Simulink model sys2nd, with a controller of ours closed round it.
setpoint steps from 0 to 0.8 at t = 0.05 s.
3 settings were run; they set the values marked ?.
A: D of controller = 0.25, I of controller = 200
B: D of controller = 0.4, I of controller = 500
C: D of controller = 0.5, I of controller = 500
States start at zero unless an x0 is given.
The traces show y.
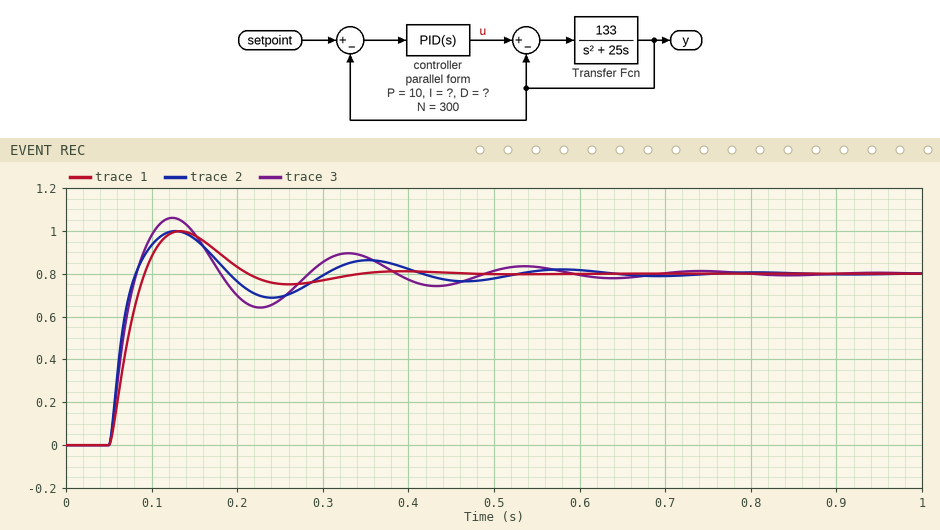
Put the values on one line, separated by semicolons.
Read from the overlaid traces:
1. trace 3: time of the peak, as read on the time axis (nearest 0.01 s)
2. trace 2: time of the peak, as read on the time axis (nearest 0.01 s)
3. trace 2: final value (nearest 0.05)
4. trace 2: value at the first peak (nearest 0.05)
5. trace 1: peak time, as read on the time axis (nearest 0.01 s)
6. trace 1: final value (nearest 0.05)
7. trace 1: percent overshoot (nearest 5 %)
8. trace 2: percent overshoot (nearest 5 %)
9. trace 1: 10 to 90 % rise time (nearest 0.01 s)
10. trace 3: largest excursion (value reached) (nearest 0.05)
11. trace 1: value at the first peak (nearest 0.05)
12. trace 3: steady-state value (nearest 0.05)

0.12 s; 0.13 s; 0.80; 1.00; 0.13 s; 0.80; 25 %; 25 %; 0.03 s; 1.05; 1.00; 0.80
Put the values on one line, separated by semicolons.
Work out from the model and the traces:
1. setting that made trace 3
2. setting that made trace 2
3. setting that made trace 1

B; C; A
